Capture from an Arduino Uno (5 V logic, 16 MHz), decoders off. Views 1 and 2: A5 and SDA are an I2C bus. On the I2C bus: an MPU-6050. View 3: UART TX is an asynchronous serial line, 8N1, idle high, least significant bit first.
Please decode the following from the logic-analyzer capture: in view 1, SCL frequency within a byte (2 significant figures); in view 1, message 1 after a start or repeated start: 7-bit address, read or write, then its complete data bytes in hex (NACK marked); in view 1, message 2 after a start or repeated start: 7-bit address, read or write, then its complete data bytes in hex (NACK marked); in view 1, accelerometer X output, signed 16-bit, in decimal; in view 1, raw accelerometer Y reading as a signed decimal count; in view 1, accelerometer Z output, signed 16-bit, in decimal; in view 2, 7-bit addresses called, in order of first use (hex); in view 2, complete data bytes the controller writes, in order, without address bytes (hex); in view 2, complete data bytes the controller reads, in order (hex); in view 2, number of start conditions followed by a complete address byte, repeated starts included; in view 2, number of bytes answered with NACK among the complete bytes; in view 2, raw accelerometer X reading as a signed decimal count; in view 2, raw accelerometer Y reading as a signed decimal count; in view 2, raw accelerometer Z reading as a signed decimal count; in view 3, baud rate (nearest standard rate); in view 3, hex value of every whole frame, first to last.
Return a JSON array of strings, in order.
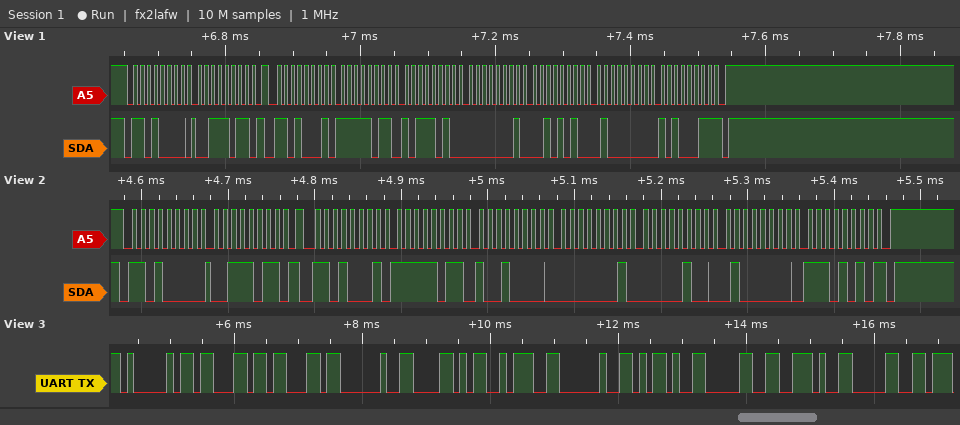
["100 kHz", "0x68 write: 3B", "0x68 read: FB BA 01 2A 40 A3 NACK", "-1094", "298", "16547", "0x68", "3B", "FB 90 01 04 40 EA", "2", "1", "-1136", "260", "16618", "9600 baud", "41 63 63 20 58 3A 20 2D 30 2E 30"]
